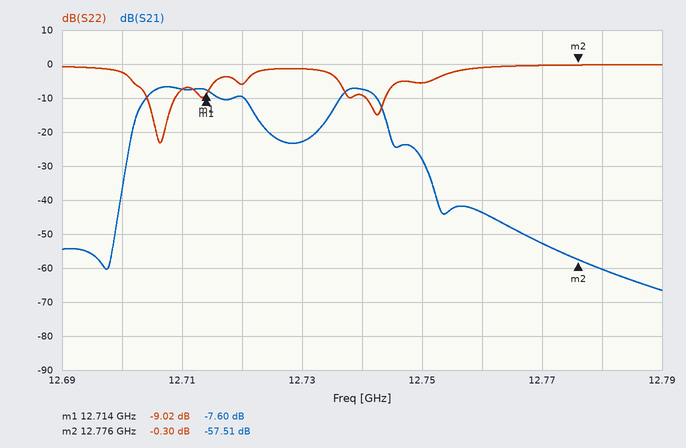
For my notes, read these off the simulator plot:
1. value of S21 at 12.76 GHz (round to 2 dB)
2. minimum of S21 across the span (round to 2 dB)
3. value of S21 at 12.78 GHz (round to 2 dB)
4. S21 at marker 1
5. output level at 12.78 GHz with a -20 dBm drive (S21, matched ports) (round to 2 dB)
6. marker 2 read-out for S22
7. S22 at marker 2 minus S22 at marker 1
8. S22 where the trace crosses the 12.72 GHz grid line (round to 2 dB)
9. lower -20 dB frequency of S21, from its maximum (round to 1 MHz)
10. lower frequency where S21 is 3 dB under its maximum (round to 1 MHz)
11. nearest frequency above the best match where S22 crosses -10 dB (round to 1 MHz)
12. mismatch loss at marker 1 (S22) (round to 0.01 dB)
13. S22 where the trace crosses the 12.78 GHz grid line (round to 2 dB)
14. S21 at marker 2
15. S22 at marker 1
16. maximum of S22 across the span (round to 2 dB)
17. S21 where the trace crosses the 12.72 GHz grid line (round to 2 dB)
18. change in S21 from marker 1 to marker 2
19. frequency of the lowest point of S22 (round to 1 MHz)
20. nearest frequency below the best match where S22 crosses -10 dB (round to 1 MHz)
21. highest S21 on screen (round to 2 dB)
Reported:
-44 dB
-66 dB
-60 dB
-7.60 dB
-80 dBm
-0.30 dB
8.72 dB
-6 dB
12.701 GHz
12.704 GHz
12.709 GHz
0.58 dB
0 dB
-57.51 dB
-9.02 dB
0 dB
-10 dB
-49.91 dB
12.706 GHz
12.704 GHz
-6 dB
